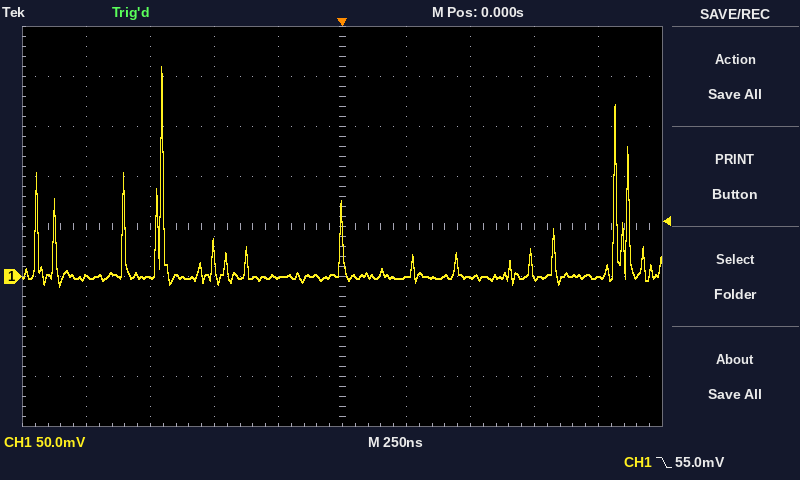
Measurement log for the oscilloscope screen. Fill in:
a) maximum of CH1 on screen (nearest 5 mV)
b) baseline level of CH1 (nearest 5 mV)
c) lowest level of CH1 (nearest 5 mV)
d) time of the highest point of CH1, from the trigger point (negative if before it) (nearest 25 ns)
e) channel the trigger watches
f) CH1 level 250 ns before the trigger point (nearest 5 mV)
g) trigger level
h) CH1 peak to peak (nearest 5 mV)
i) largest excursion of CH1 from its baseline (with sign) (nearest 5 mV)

210 mV
0 mV
-10 mV
-700 ns
CH1
0 mV
55.0 mV
220 mV
+210 mV
